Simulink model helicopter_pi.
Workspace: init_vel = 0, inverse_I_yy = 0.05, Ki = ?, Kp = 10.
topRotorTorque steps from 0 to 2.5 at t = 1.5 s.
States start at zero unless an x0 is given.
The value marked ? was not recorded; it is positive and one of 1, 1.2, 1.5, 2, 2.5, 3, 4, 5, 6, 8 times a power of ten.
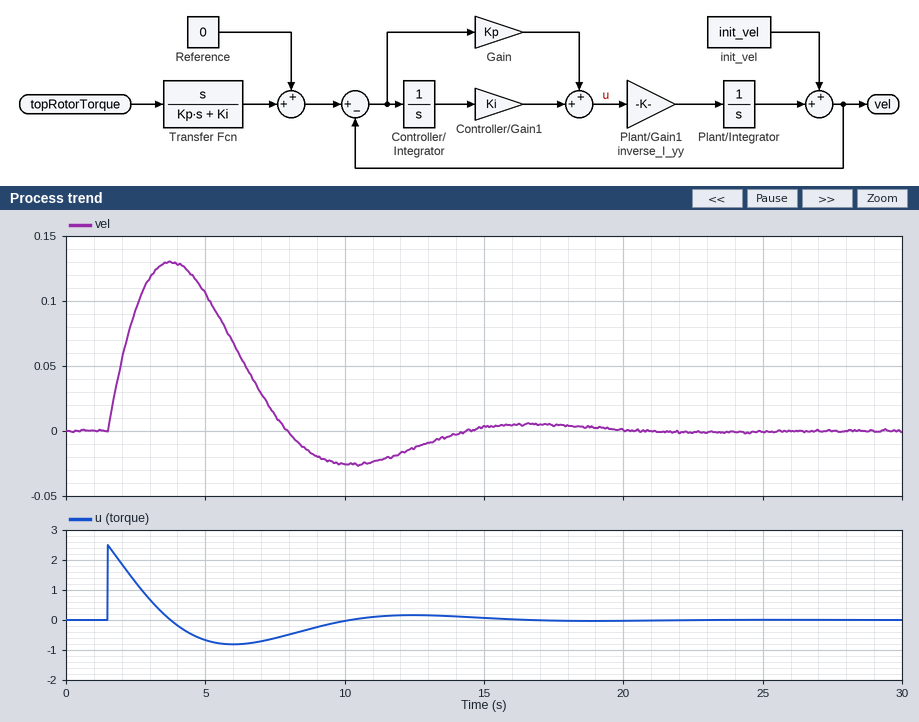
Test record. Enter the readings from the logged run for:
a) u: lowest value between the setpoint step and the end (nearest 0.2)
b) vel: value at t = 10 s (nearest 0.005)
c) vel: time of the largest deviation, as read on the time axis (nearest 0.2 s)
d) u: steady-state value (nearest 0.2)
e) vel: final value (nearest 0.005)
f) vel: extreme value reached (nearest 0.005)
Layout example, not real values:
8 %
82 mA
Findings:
-0.8
-0.025
3.8 s
0.0
0.000
0.130
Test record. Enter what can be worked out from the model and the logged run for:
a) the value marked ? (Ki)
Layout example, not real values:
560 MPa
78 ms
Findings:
6
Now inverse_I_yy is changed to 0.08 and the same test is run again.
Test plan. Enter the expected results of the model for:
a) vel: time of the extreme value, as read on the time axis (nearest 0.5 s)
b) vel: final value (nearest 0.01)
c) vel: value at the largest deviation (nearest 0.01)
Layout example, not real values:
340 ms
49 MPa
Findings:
3.0 s
0.00
0.15
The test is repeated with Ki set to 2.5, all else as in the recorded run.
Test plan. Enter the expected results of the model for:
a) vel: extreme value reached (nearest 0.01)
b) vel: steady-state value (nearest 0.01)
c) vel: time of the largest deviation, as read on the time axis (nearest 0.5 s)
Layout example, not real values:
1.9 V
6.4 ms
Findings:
0.16
0.00
4.5 s
